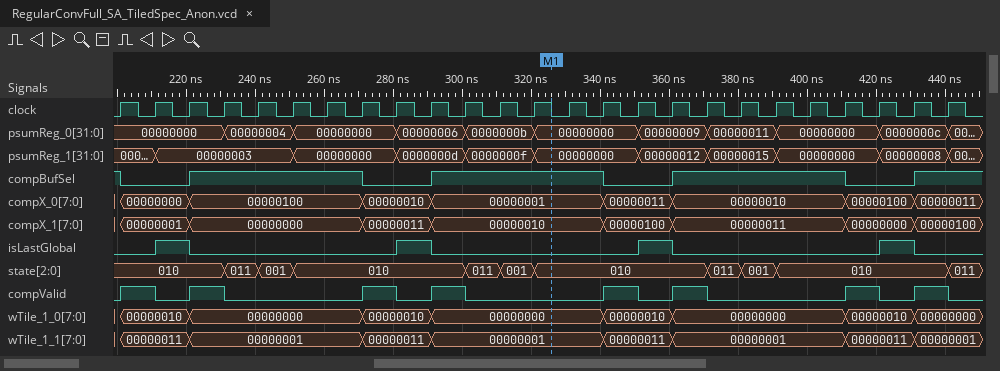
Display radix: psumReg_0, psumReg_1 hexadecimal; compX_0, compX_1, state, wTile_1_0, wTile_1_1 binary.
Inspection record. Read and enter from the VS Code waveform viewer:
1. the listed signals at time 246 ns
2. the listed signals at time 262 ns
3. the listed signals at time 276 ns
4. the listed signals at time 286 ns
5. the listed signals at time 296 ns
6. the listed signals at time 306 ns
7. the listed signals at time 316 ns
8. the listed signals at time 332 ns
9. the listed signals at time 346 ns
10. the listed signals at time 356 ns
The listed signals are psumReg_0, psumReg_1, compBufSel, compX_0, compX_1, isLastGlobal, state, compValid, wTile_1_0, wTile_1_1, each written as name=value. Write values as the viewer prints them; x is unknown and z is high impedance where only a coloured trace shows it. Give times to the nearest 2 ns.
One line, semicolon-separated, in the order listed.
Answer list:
psumReg_0=00000004, psumReg_1=00000003, compBufSel=1, compX_0=00000100, compX_1=00000000, isLastGlobal=0, state=001, compValid=0, wTile_1_0=00000000, wTile_1_1=00000001; psumReg_0=00000000, psumReg_1=00000000, compBufSel=1, compX_0=00000100, compX_1=00000000, isLastGlobal=0, state=010, compValid=0, wTile_1_0=00000000, wTile_1_1=00000001; psumReg_0=00000000, psumReg_1=00000000, compBufSel=0, compX_0=00000010, compX_1=00000011, isLastGlobal=0, state=010, compValid=1, wTile_1_0=00000010, wTile_1_1=00000011; psumReg_0=00000006, psumReg_1=0000000d, compBufSel=0, compX_0=00000010, compX_1=00000011, isLastGlobal=1, state=010, compValid=0, wTile_1_0=00000010, wTile_1_1=00000011; psumReg_0=00000006, psumReg_1=0000000d, compBufSel=1, compX_0=00000001, compX_1=00000010, isLastGlobal=0, state=010, compValid=1, wTile_1_0=00000000, wTile_1_1=00000001; psumReg_0=0000000b, psumReg_1=0000000f, compBufSel=1, compX_0=00000001, compX_1=00000010, isLastGlobal=0, state=011, compValid=0, wTile_1_0=00000000, wTile_1_1=00000001; psumReg_0=0000000b, psumReg_1=0000000f, compBufSel=1, compX_0=00000001, compX_1=00000010, isLastGlobal=0, state=001, compValid=0, wTile_1_0=00000000, wTile_1_1=00000001; psumReg_0=00000000, psumReg_1=00000000, compBufSel=1, compX_0=00000001, compX_1=00000010, isLastGlobal=0, state=010, compValid=0, wTile_1_0=00000000, wTile_1_1=00000001; psumReg_0=00000000, psumReg_1=00000000, compBufSel=0, compX_0=00000011, compX_1=00000100, isLastGlobal=0, state=010, compValid=1, wTile_1_0=00000010, wTile_1_1=00000011; psumReg_0=00000009, psumReg_1=00000012, compBufSel=0, compX_0=00000011, compX_1=00000100, isLastGlobal=1, state=010, compValid=0, wTile_1_0=00000010, wTile_1_1=00000011
